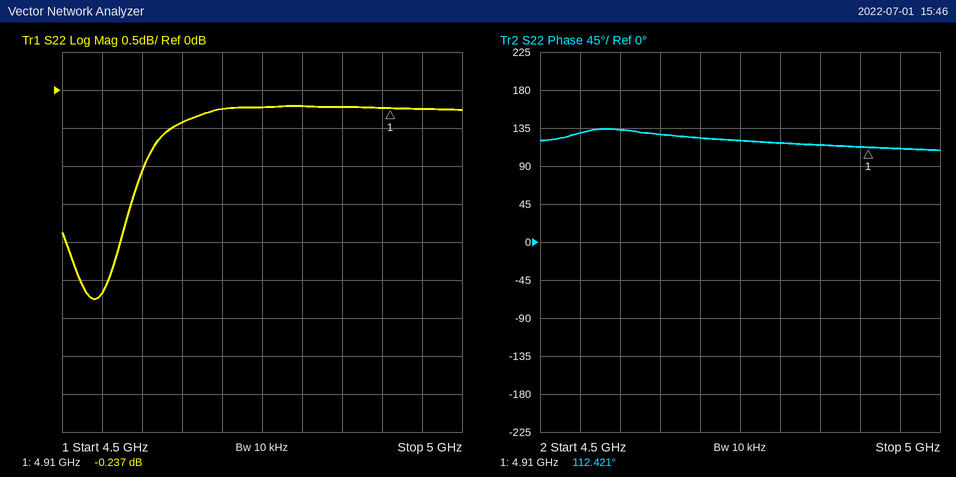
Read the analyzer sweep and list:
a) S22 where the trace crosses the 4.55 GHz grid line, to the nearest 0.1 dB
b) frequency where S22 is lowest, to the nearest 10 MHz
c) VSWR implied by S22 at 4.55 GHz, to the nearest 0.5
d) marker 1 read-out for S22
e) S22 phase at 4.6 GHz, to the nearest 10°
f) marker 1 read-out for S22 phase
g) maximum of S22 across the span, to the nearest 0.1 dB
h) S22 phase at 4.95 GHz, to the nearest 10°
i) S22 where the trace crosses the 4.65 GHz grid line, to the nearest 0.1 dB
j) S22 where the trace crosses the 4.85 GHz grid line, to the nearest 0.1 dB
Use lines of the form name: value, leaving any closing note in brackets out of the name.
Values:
S22 where the trace crosses the 4.55 GHz grid line, to the nearest 0.1 dB: -2.7 dB
frequency where S22 is lowest, to the nearest 10 MHz: 4.54 GHz
VSWR implied by S22 at 4.55 GHz, to the nearest 0.5: 6.5
marker 1 read-out for S22: -0.237 dB
S22 phase at 4.6 GHz, to the nearest 10°: 130°
marker 1 read-out for S22 phase: 112.421°
maximum of S22 across the span, to the nearest 0.1 dB: -0.2 dB
S22 phase at 4.95 GHz, to the nearest 10°: 110°
S22 where the trace crosses the 4.65 GHz grid line, to the nearest 0.1 dB: -0.4 dB
S22 where the trace crosses the 4.85 GHz grid line, to the nearest 0.1 dB: -0.2 dB
